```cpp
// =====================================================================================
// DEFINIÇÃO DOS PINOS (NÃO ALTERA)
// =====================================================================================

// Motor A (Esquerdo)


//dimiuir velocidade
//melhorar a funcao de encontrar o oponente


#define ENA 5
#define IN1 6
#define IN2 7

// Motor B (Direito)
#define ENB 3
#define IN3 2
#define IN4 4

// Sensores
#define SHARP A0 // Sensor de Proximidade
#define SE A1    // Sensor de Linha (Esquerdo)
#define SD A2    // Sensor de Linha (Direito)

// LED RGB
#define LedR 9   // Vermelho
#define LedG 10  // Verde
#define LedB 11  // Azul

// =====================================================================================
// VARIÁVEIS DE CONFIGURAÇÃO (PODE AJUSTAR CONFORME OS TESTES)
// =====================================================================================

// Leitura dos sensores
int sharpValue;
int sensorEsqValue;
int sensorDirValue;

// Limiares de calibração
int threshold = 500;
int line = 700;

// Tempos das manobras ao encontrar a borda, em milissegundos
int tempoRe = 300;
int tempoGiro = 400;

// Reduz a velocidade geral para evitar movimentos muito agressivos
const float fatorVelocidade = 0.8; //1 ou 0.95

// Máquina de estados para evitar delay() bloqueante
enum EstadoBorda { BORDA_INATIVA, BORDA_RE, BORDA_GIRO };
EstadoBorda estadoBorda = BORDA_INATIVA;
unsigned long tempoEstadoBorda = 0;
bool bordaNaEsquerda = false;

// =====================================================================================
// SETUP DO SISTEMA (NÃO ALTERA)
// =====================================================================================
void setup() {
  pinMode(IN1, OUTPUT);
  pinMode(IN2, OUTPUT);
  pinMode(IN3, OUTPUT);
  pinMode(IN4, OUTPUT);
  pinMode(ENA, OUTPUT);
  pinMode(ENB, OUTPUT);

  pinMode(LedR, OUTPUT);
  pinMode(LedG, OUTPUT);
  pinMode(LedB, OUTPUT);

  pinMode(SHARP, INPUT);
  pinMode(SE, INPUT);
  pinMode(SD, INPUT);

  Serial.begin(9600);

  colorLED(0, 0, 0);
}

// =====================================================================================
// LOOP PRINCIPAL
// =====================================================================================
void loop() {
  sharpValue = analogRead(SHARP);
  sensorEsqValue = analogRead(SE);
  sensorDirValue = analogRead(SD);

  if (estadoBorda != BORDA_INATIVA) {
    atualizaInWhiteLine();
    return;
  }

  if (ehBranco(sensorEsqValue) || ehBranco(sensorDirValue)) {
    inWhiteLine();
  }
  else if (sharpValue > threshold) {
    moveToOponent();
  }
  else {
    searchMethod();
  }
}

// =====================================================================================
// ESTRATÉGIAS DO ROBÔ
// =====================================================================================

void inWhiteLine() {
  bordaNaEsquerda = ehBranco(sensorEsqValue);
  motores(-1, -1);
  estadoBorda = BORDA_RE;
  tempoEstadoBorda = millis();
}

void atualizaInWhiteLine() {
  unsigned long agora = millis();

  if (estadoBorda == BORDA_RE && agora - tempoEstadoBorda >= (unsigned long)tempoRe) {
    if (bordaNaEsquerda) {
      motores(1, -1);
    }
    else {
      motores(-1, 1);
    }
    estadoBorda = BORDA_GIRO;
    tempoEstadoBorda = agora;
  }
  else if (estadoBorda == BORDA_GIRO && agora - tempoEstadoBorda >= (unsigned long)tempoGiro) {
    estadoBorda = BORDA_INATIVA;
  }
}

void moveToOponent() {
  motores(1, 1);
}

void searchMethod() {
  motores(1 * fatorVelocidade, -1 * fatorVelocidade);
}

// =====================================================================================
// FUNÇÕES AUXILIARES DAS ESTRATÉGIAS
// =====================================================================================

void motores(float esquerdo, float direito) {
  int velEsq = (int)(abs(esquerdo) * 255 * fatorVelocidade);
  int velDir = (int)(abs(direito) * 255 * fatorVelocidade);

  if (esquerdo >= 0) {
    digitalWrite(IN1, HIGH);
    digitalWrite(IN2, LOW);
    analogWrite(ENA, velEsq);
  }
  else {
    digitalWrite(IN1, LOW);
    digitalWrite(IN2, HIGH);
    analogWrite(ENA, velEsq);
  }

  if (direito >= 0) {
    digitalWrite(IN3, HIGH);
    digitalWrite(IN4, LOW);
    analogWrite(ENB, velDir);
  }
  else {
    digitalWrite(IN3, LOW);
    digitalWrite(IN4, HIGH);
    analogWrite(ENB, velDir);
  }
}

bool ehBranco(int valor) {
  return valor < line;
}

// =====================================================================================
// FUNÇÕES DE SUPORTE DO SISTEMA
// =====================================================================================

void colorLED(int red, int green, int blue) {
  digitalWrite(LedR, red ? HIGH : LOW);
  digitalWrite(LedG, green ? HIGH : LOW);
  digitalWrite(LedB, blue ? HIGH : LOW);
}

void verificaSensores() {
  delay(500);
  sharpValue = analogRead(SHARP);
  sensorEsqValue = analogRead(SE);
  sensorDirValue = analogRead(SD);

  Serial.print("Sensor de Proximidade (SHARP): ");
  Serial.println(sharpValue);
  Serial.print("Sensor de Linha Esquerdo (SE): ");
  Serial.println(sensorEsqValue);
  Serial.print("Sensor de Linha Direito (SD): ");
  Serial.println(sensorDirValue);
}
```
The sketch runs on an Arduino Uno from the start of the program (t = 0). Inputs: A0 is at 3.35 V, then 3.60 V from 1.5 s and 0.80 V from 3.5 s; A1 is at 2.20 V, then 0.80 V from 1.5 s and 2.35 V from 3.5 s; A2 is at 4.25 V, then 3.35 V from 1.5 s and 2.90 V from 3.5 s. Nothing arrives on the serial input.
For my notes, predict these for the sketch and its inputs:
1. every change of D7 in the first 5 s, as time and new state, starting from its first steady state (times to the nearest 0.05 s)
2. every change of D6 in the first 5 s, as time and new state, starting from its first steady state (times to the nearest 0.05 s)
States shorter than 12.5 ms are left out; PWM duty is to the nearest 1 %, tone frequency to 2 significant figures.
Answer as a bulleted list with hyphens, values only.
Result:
- 0 s high; 0.3 s low; 0.7 s high; 1 s low; 1.4 s high; 1.7 s low; 2.1 s high; 2.4 s low; 2.8 s high; 3.1 s low; 3.5 s high; 3.8 s low; 4.2 s high; 4.5 s low; 4.9 s high
- 0 s low; 0.3 s high; 0.7 s low; 1 s high; 1.4 s low; 1.7 s high; 2.1 s low; 2.4 s high; 2.8 s low; 3.1 s high; 3.5 s low; 3.8 s high; 4.2 s low; 4.5 s high; 4.9 s low
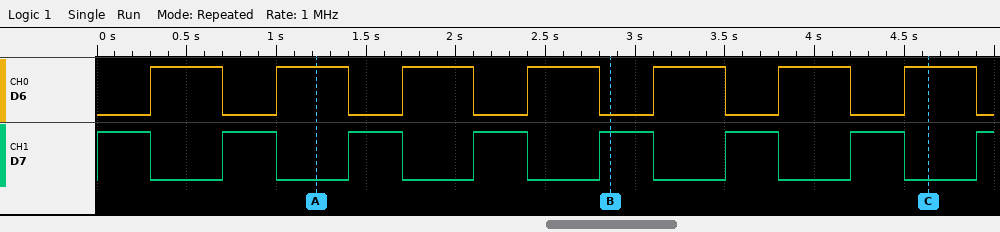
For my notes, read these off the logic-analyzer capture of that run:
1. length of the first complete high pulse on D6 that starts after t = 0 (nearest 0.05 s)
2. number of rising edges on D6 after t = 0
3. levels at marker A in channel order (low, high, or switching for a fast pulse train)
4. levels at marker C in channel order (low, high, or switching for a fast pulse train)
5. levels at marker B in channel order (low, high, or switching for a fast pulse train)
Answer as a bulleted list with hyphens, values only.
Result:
- 0.40 s
- 7
- D6 high, D7 low
- D6 high, D7 low
- D6 low, D7 high
